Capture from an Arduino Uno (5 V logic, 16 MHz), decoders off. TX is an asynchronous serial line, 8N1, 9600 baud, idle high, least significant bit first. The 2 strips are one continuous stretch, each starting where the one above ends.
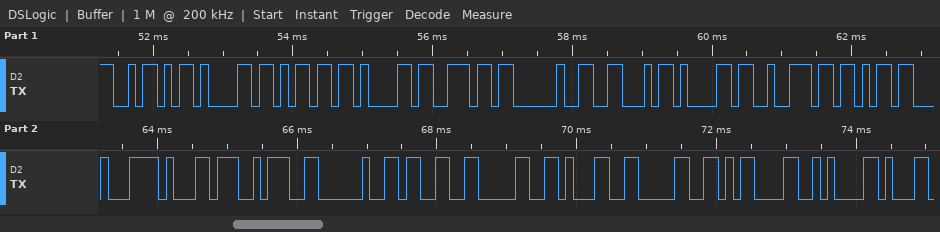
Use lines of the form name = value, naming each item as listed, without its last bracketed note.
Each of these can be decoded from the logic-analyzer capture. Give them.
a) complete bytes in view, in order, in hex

complete bytes in view, in order, in hex = 0x5A 0x61 0x6D 0x61 0x6E 0x20 0x46 0x61 0x72 0x6B 0xC4 0xB1 0x3A 0x20 0x33 0x30 0x31 0x30 0x0D 0x0A
